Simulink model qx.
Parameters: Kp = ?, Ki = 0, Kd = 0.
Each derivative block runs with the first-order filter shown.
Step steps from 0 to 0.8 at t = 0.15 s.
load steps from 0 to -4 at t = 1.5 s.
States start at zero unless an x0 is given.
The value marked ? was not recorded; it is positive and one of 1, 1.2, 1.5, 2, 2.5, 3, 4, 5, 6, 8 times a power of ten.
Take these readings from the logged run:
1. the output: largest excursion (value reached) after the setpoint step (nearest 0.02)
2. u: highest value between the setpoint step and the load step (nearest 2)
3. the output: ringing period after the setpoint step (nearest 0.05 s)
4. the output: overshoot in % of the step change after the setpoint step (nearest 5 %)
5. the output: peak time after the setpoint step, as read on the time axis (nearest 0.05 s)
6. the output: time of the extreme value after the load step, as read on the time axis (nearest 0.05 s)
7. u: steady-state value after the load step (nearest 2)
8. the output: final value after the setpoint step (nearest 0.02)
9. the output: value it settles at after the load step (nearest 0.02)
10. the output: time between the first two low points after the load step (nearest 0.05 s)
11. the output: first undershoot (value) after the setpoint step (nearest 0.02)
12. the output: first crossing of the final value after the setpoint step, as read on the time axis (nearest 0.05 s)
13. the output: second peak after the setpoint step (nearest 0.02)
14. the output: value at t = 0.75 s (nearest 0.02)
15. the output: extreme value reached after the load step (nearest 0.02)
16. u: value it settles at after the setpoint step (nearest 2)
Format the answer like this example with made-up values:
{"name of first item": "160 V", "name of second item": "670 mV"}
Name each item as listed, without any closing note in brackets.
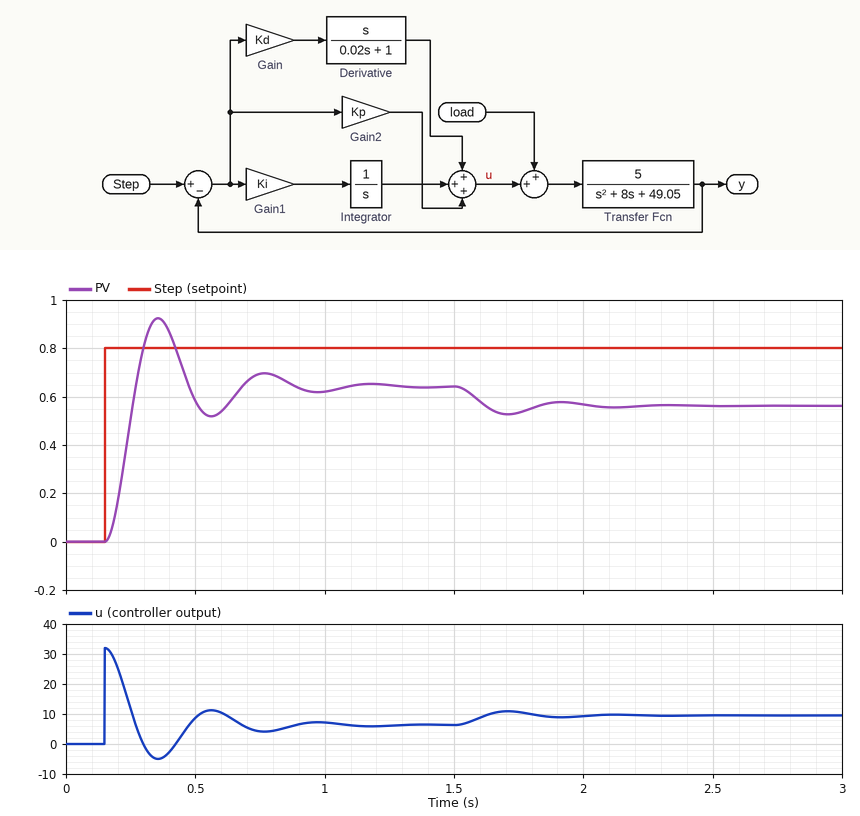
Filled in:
{"the output: largest excursion (value reached) after the setpoint step": "0.92", "u: highest value between the setpoint step and the load step": "32", "the output: ringing period after the setpoint step": "0.40 s", "the output: overshoot in % of the step change after the setpoint step": "45 %", "the output: peak time after the setpoint step, as read on the time axis": "0.35 s", "the output: time of the extreme value after the load step, as read on the time axis": "1.70 s", "u: steady-state value after the load step": "10", "the output: final value after the setpoint step": "0.64", "the output: value it settles at after the load step": "0.56", "the output: time between the first two low points after the load step": "0.40 s", "the output: first undershoot (value) after the setpoint step": "0.52", "the output: first crossing of the final value after the setpoint step, as read on the time axis": "0.25 s", "the output: second peak after the setpoint step": "0.70", "the output: value at t = 0.75 s": "0.70", "the output: extreme value reached after the load step": "0.52", "u: value it settles at after the setpoint step": "6"}
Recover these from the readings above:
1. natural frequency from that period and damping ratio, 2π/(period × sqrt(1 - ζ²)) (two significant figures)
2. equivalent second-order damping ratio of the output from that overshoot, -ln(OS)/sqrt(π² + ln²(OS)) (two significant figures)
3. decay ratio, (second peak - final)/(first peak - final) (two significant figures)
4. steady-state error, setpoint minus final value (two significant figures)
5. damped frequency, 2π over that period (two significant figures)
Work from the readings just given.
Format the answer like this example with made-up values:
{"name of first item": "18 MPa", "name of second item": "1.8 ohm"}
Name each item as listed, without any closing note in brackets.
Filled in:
{"natural frequency from that period and damping ratio, 2π/(period × sqrt(1 - ζ²))": "16 rad/s", "equivalent second-order damping ratio of the output from that overshoot, -ln(OS)/sqrt(π² + ln²(OS))": "0.25", "decay ratio, (second peak - final)/(first peak - final)": "0.21", "steady-state error, setpoint minus final value": "0.16", "damped frequency, 2π over that period": "16 rad/s"}
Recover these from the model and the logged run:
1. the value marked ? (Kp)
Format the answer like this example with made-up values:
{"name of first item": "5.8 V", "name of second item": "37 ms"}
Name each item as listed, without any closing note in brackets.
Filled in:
{"the value marked ?": "40"}
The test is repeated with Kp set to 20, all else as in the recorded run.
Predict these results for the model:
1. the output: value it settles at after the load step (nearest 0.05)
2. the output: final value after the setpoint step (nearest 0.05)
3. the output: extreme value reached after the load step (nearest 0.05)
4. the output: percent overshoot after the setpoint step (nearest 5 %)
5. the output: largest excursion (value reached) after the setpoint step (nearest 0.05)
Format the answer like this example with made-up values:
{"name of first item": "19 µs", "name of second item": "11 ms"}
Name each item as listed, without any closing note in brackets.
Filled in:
{"the output: value it settles at after the load step": "0.40", "the output: final value after the setpoint step": "0.55", "the output: extreme value reached after the load step": "0.35", "the output: percent overshoot after the setpoint step": "35 %", "the output: largest excursion (value reached) after the setpoint step": "0.70"}
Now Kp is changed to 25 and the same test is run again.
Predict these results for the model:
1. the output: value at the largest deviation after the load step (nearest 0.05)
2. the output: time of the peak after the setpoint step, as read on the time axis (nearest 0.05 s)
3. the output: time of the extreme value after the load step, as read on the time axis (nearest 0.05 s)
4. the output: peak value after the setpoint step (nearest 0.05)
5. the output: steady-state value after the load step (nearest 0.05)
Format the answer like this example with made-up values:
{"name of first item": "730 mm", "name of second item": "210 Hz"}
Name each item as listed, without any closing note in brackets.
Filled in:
{"the output: value at the largest deviation after the load step": "0.40", "the output: time of the peak after the setpoint step, as read on the time axis": "0.40 s", "the output: time of the extreme value after the load step, as read on the time axis": "1.75 s", "the output: peak value after the setpoint step": "0.80", "the output: steady-state value after the load step": "0.45"}
